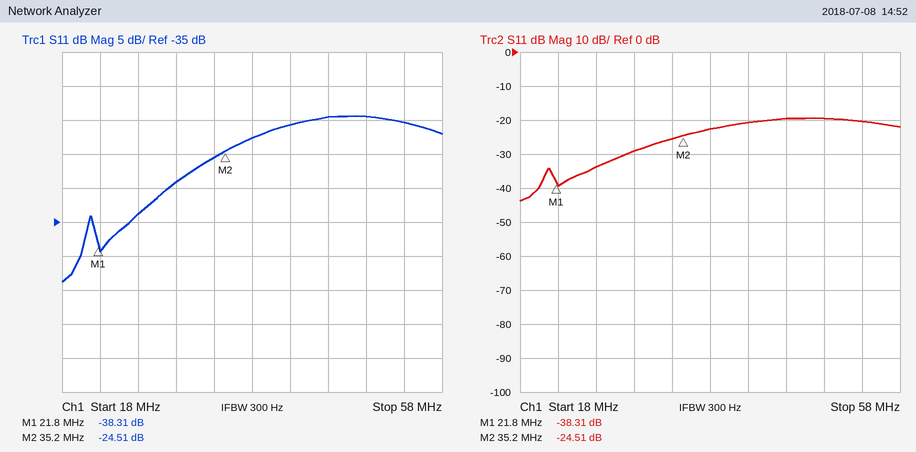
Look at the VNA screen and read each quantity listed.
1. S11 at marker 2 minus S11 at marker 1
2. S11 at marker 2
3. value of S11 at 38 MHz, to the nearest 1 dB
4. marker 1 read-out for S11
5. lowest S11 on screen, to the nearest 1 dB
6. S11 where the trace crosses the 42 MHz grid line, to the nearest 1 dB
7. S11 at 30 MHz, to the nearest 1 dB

13.80 dB
-24.51 dB
-23 dB
-38.31 dB
-44 dB
-21 dB
-29 dB
